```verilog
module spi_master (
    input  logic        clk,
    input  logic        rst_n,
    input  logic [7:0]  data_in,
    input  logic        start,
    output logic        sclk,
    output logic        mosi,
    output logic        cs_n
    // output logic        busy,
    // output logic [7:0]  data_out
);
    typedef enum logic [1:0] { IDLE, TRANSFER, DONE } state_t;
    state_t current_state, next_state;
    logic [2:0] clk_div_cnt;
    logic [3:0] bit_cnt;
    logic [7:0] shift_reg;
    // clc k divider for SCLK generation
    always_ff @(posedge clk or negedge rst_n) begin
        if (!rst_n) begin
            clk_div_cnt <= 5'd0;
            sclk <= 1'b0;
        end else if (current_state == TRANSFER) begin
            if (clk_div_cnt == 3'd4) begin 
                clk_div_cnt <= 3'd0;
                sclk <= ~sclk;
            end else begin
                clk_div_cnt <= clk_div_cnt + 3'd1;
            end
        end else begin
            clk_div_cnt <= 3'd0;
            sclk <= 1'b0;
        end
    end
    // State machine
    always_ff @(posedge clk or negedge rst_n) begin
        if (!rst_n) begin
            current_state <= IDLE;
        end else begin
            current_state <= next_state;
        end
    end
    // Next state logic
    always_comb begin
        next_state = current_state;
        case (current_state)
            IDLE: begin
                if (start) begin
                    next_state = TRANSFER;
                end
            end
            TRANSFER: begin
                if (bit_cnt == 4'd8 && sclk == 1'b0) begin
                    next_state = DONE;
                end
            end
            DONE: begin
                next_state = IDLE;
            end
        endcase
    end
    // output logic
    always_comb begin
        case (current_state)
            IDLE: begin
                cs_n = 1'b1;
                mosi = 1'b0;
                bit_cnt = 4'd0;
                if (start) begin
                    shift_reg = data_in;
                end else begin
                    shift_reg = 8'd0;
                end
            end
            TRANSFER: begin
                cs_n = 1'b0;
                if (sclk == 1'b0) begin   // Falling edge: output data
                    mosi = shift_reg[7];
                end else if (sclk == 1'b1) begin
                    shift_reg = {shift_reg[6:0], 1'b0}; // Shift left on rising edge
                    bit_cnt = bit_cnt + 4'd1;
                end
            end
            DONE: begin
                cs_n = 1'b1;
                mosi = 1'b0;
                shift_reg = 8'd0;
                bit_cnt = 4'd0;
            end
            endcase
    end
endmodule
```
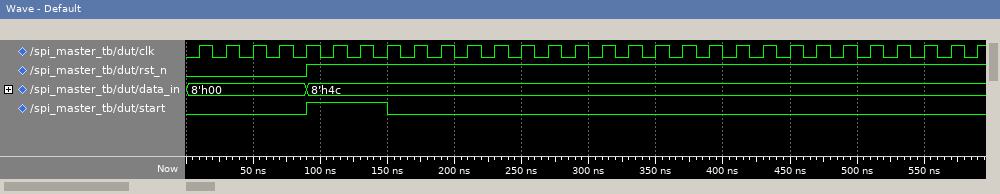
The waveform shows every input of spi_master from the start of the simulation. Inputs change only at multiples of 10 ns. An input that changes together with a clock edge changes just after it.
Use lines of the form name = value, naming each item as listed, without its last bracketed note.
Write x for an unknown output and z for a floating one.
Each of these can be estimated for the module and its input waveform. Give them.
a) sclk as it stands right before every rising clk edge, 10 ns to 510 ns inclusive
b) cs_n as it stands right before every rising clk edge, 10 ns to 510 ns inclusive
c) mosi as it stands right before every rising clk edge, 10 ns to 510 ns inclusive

sclk as it stands right before every rising clk edge, 10 ns to 510 ns inclusive = 0 0 0 0 0 0 0 0 0 0 0 1 1 1 1 1 0 0 0 0 0 1 1 1 1 1
cs_n as it stands right before every rising clk edge, 10 ns to 510 ns inclusive = 1 1 1 1 1 1 0 0 0 0 0 0 0 0 0 0 0 0 0 0 0 0 0 0 0 0
mosi as it stands right before every rising clk edge, 10 ns to 510 ns inclusive = 0 0 0 0 0 0 0 0 0 0 0 0 0 0 0 0 1 1 1 1 1 1 1 1 1 1
